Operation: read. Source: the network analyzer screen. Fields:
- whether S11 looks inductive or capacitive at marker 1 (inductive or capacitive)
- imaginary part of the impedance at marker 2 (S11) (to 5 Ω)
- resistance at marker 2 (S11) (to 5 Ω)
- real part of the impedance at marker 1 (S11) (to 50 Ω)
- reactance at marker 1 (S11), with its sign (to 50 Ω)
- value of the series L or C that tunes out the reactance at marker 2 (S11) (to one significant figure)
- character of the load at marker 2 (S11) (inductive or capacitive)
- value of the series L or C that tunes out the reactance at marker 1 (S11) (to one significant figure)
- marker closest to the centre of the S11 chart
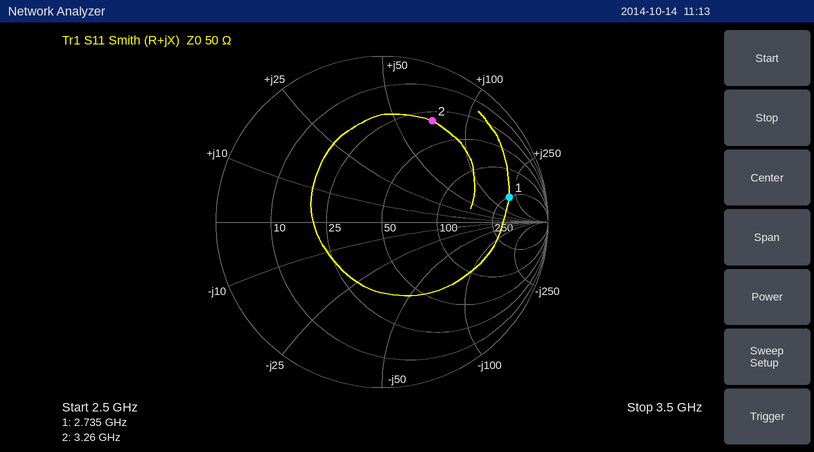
inductive
+70 Ω
30 Ω
250 Ω
+200 Ω
700 fF
inductive
300 fF
marker 2
